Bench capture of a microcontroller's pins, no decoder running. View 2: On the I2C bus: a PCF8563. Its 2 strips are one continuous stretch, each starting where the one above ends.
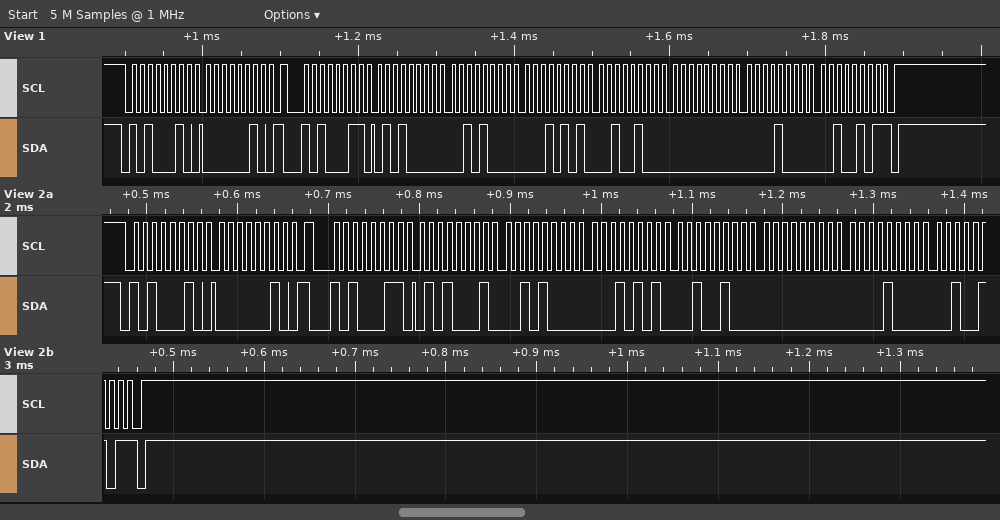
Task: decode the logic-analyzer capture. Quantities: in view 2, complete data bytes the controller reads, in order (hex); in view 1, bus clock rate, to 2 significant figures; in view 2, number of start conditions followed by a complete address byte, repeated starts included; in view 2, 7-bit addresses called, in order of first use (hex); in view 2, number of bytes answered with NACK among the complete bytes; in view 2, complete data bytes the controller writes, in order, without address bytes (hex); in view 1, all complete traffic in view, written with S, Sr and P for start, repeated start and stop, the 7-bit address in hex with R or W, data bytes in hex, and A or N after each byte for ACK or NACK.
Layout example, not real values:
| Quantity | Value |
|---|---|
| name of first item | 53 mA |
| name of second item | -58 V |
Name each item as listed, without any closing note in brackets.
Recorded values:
| Quantity | Value |
|---|---|
| in view 2, complete data bytes the controller reads, in order | 51 28 15 24 00 08 25 |
| in view 1, bus clock rate, to 2 significant figures | 100 kHz |
| in view 2, number of start conditions followed by a complete address byte, repeated starts included | 2 |
| in view 2, 7-bit addresses called, in order of first use | 0x51 |
| in view 2, number of bytes answered with NACK among the complete bytes | 1 |
| in view 2, complete data bytes the controller writes, in order, without address bytes | 02 |
| in view 1, all complete traffic in view, written with S, Sr and P for start, repeated start and stop, the 7-bit address in hex with R or W, data bytes in hex, and A or N after each byte for ACK or NACK | S 51W A 02 A Sr 51R A 50 A 28 A 15 A 24 A 00 A 08 A 25 N P |
